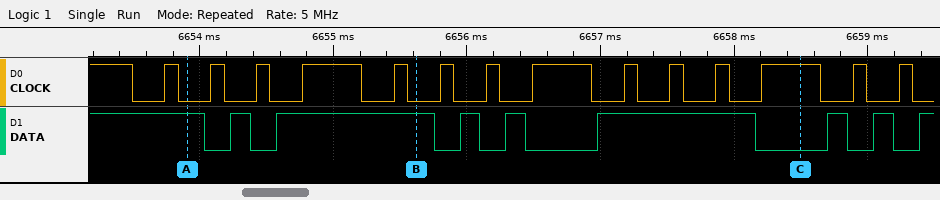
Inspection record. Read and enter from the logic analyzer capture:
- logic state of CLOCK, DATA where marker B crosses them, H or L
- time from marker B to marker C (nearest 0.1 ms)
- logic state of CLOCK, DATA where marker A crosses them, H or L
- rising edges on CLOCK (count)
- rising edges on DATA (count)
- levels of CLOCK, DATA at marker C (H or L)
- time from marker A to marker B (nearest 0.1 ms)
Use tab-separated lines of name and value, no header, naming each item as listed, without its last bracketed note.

logic state of CLOCK, DATA where marker B crosses them, H or L	CLOCK=L, DATA=H
time from marker B to marker C	2.9 ms
logic state of CLOCK, DATA where marker A crosses them, H or L	CLOCK=L, DATA=H
rising edges on CLOCK	14
rising edges on DATA	8
levels of CLOCK, DATA at marker C	CLOCK=H, DATA=L
time from marker A to marker B	1.7 ms
